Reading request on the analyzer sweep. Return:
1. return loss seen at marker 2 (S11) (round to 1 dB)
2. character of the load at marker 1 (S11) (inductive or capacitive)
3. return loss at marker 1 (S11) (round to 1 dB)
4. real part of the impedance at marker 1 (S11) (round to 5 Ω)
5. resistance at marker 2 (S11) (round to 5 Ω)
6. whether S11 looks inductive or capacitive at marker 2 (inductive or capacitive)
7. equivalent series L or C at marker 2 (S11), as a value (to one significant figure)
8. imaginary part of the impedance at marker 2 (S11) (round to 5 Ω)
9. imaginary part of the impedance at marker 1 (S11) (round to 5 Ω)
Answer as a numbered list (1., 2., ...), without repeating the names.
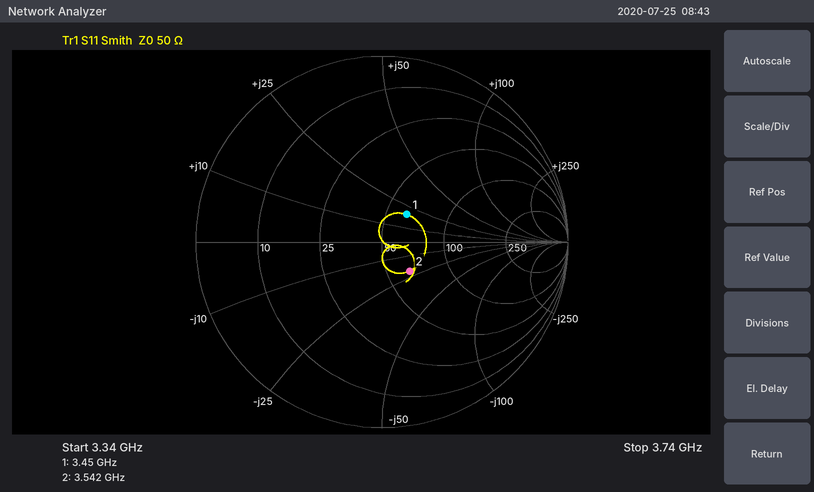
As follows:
1. 13 dB
2. inductive
3. 14 dB
4. 60 Ω
5. 65 Ω
6. capacitive
7. 2 pF
8. -20 Ω
9. +20 Ω
